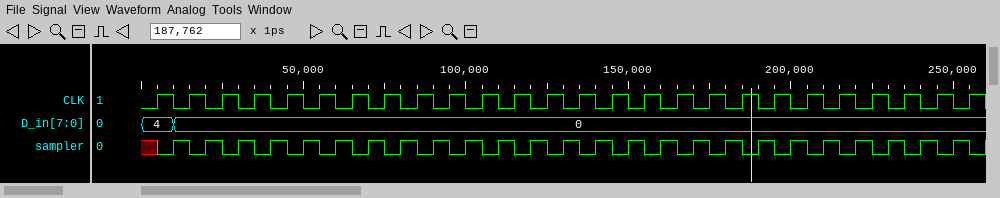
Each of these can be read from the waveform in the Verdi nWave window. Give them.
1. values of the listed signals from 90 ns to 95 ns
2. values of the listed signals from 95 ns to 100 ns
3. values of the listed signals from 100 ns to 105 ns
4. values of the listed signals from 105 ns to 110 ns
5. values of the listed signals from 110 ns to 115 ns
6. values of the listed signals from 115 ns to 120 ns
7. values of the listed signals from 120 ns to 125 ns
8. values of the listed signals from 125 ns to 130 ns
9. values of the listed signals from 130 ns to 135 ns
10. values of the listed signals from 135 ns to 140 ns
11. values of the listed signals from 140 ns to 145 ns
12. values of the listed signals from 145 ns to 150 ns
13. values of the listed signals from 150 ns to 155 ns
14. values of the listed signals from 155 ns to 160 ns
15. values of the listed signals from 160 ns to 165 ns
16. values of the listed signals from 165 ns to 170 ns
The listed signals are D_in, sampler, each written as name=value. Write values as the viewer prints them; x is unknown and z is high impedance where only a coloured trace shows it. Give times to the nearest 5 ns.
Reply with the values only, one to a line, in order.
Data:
D_in=0, sampler=1
D_in=0, sampler=0
D_in=0, sampler=1
D_in=0, sampler=0
D_in=0, sampler=1
D_in=0, sampler=0
D_in=0, sampler=1
D_in=0, sampler=0
D_in=0, sampler=1
D_in=0, sampler=0
D_in=0, sampler=1
D_in=0, sampler=0
D_in=0, sampler=1
D_in=0, sampler=0
D_in=0, sampler=1
D_in=0, sampler=0
